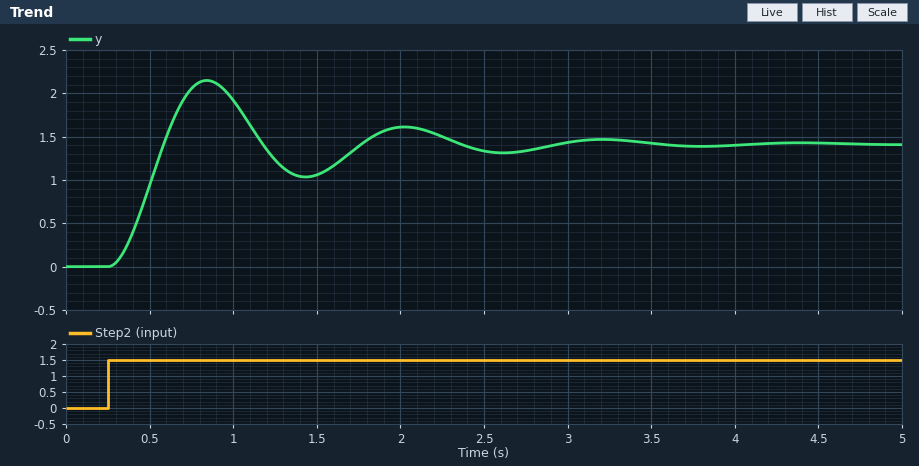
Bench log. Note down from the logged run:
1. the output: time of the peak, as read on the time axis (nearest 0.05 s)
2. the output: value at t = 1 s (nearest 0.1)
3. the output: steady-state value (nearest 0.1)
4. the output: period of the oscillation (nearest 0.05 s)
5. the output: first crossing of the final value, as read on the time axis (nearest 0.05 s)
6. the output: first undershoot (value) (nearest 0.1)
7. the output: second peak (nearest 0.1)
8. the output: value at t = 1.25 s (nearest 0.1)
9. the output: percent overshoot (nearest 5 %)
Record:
0.85 s
1.9
1.4
1.20 s
0.60 s
1.0
1.6
1.2
50 %
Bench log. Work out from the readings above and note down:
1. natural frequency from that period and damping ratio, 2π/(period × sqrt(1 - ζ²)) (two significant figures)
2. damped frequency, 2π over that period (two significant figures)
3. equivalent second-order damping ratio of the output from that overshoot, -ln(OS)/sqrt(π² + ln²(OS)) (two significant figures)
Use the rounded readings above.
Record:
5.4 rad/s
5.2 rad/s
0.22
